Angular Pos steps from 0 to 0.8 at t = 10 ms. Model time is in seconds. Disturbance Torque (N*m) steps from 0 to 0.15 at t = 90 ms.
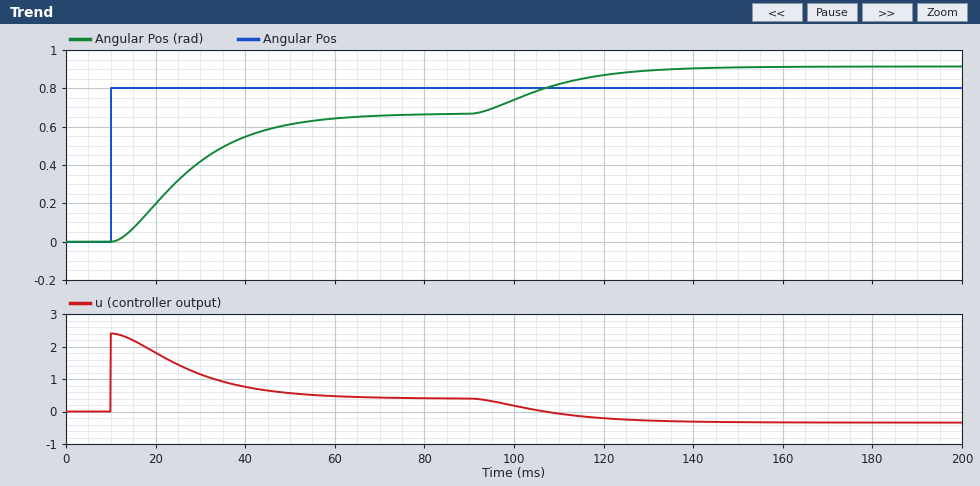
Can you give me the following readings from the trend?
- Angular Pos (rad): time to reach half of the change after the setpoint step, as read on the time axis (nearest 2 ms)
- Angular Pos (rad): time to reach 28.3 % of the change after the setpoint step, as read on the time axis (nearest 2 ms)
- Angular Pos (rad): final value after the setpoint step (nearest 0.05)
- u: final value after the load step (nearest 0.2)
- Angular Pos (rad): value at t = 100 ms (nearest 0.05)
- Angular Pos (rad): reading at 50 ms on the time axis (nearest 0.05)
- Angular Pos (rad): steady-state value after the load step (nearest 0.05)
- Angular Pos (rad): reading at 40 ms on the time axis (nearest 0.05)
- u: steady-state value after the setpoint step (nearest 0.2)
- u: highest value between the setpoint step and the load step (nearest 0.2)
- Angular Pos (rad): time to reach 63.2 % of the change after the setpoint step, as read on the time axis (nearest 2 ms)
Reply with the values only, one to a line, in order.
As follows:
26 ms
20 ms
0.65
-0.4
0.75
0.60
0.90
0.55
0.4
2.4
30 ms
